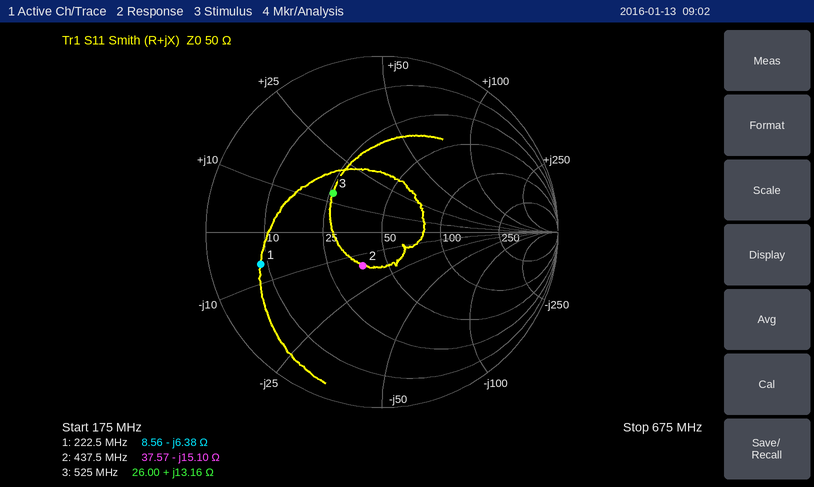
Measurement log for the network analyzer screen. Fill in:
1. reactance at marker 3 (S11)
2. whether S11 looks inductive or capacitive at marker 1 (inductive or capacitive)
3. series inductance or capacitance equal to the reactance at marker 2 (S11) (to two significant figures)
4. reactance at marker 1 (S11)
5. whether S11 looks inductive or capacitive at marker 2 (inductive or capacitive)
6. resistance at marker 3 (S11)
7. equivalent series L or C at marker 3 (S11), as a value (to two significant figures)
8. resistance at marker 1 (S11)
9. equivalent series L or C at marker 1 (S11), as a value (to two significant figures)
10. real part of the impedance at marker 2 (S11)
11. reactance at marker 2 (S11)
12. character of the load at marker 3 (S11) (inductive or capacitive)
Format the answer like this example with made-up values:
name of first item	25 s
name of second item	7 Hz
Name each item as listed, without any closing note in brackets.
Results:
reactance at marker 3	+13.16 Ω
whether S11 looks inductive or capacitive at marker 1	capacitive
series inductance or capacitance equal to the reactance at marker 2 (S11)	24 pF
reactance at marker 1	-6.38 Ω
whether S11 looks inductive or capacitive at marker 2	capacitive
resistance at marker 3	26.00 Ω
equivalent series L or C at marker 3 (S11), as a value	4.0 nH
resistance at marker 1	8.56 Ω
equivalent series L or C at marker 1 (S11), as a value	110 pF
real part of the impedance at marker 2	37.57 Ω
reactance at marker 2	-15.10 Ω
character of the load at marker 3 (S11)	inductive
